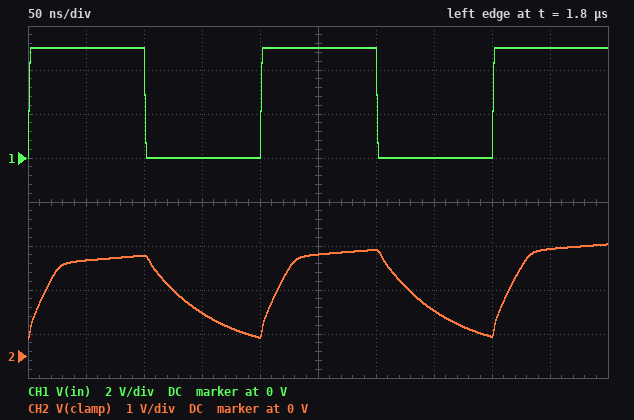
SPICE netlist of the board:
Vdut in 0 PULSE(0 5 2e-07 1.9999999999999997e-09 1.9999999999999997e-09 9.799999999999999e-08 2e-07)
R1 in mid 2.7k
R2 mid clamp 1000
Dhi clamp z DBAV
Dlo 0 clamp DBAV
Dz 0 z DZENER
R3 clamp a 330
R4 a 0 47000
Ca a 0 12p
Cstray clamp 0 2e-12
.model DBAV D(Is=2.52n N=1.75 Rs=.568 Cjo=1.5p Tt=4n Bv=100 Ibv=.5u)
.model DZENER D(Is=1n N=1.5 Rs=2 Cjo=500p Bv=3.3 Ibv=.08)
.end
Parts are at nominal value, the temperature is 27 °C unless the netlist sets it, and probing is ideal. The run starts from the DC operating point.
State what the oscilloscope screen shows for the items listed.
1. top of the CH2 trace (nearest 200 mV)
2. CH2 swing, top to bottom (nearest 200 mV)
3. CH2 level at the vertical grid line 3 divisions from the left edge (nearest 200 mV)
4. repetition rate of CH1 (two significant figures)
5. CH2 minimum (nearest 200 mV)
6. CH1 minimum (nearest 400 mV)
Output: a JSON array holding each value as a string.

["2.6 V", "2.2 V", "1.0 V", "5.0 MHz", "400 mV", "0 V"]
